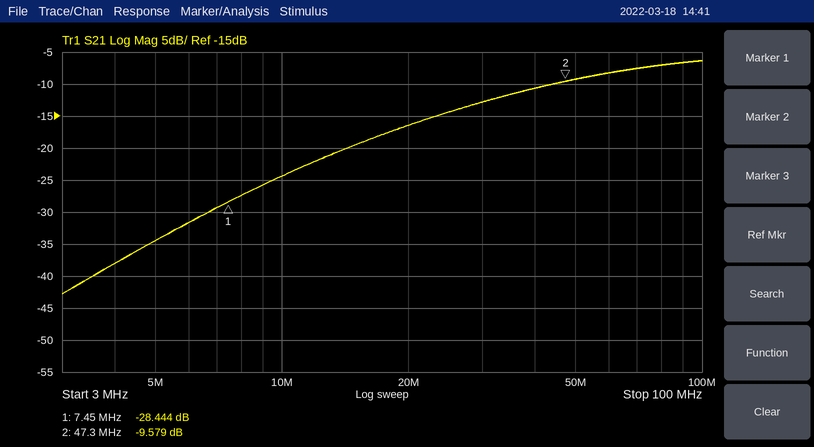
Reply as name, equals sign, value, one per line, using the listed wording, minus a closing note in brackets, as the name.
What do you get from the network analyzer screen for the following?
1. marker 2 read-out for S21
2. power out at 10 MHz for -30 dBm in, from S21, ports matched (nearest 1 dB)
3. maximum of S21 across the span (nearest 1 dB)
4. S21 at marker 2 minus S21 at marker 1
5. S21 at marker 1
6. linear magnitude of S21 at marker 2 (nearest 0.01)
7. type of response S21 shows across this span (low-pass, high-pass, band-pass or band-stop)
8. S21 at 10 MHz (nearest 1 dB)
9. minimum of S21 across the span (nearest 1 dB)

marker 2 read-out for S21 = -9.579 dB
power out at 10 MHz for -30 dBm in, from S21, ports matched = -54 dBm
maximum of S21 across the span = -6 dB
S21 at marker 2 minus S21 at marker 1 = 18.865 dB
S21 at marker 1 = -28.444 dB
linear magnitude of S21 at marker 2 = 0.33
type of response S21 shows across this span = high-pass
S21 at 10 MHz = -24 dB
minimum of S21 across the span = -43 dB
